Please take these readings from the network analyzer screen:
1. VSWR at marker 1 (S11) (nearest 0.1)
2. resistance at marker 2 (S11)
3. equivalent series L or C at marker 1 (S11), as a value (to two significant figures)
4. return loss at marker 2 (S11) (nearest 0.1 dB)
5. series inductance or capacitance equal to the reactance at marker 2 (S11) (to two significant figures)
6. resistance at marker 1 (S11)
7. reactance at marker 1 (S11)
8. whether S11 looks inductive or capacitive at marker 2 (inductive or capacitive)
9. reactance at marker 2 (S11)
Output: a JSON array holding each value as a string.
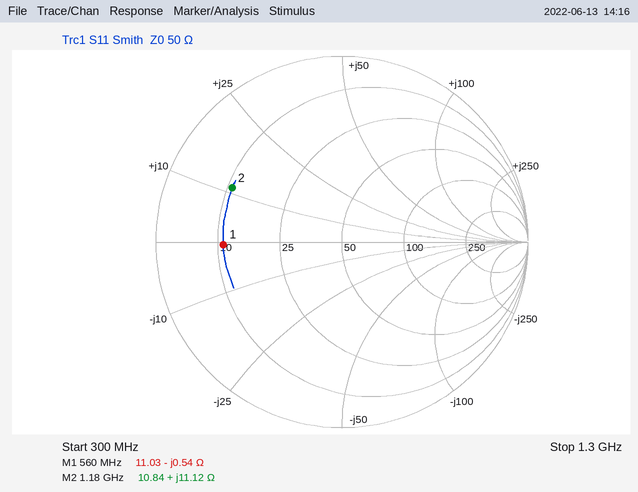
["4.5", "10.84 Ω", "530 pF", "3.6 dB", "1.5 nH", "11.03 Ω", "-0.54 Ω", "inductive", "+11.12 Ω"]
